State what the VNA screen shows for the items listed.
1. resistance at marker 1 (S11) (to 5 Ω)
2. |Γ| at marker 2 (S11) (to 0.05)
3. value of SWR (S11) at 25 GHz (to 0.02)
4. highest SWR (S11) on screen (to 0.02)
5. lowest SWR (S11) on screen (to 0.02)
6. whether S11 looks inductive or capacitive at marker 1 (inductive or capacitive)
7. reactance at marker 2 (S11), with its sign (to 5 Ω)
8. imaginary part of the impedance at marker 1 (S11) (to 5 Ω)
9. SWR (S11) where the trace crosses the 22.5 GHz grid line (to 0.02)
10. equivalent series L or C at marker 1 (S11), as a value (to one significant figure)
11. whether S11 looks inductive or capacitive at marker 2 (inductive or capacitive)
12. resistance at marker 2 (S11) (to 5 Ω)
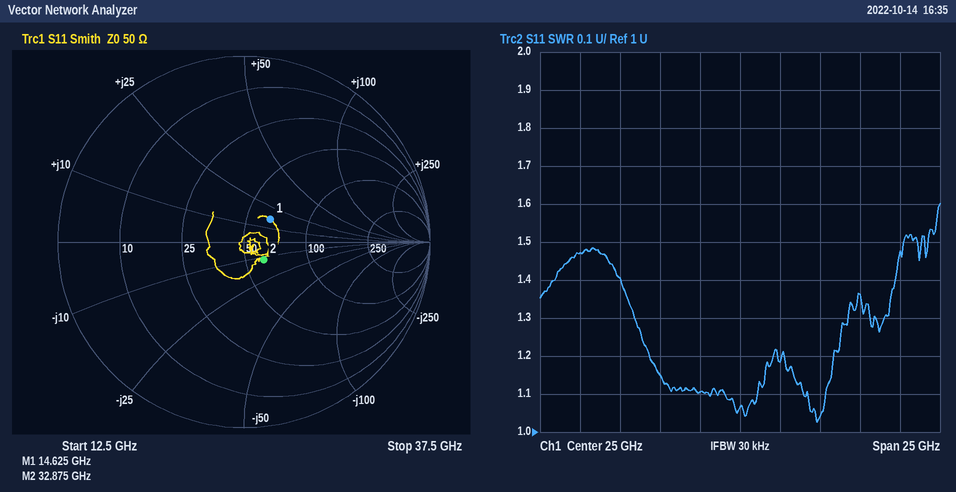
65 Ω
0.15
1.06
1.60
1.02
inductive
-10 Ω
+15 Ω
1.10
200 pH
capacitive
60 Ω
